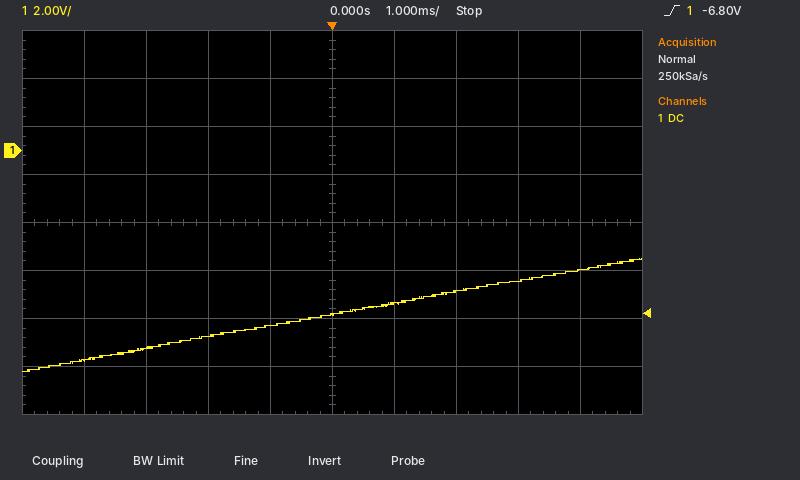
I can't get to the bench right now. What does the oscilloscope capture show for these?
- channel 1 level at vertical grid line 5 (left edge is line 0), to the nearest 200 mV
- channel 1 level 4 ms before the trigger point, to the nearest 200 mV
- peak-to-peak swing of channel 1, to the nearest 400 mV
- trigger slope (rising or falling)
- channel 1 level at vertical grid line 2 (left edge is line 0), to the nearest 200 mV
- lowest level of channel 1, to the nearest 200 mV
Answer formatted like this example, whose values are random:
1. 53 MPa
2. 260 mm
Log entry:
1. -6.8 V
2. -8.8 V
3. 4.8 V
4. rising
5. -8.2 V
6. -9.2 V
